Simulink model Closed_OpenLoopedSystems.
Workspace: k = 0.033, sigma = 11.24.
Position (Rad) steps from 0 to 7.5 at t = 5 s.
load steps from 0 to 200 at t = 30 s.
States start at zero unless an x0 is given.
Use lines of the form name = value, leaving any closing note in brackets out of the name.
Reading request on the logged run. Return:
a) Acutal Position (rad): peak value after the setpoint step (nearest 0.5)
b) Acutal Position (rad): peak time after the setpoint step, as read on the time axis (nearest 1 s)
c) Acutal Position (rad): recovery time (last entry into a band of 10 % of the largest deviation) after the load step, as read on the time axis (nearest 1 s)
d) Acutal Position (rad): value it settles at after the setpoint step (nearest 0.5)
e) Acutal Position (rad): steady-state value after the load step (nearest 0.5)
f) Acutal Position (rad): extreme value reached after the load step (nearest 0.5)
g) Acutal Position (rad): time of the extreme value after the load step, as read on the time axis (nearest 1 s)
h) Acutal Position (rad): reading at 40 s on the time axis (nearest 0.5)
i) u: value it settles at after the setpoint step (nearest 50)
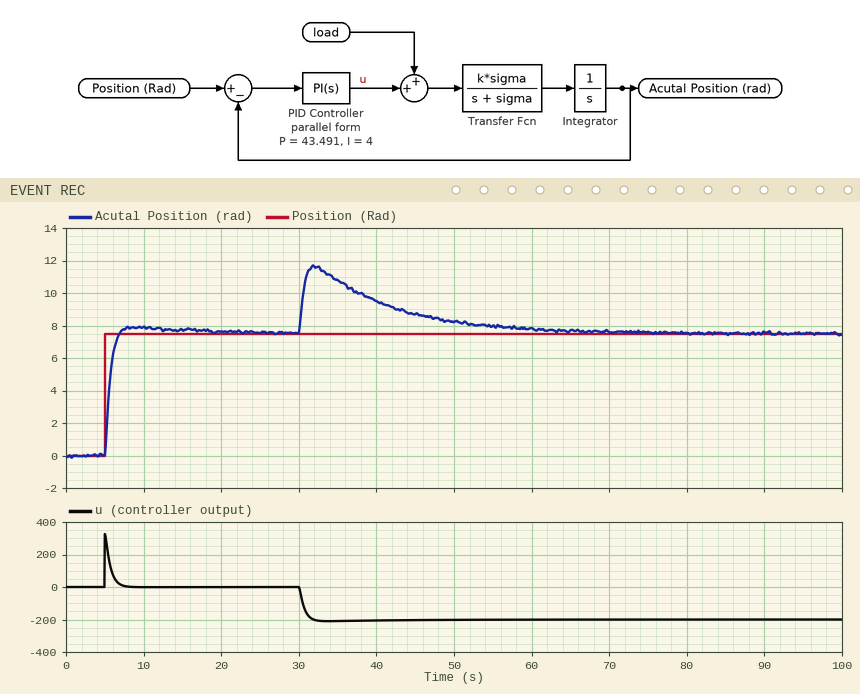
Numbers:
Acutal Position (rad): peak value after the setpoint step = 8.0
Acutal Position (rad): peak time after the setpoint step, as read on the time axis = 9 s
Acutal Position (rad): recovery time (last entry into a band of 10 % of the largest deviation) after the load step, as read on the time axis = 56 s
Acutal Position (rad): value it settles at after the setpoint step = 7.5
Acutal Position (rad): steady-state value after the load step = 7.5
Acutal Position (rad): extreme value reached after the load step = 11.5
Acutal Position (rad): time of the extreme value after the load step, as read on the time axis = 32 s
Acutal Position (rad): reading at 40 s on the time axis = 9.5
u: value it settles at after the setpoint step = 0
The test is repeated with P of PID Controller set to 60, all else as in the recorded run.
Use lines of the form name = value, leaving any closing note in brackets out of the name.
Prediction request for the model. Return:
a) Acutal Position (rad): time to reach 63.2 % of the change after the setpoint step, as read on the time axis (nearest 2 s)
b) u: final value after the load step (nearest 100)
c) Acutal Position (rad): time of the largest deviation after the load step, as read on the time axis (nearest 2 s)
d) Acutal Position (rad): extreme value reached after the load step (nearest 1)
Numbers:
Acutal Position (rad): time to reach 63.2 % of the change after the setpoint step, as read on the time axis = 6 s
u: final value after the load step = -200
Acutal Position (rad): time of the largest deviation after the load step, as read on the time axis = 32 s
Acutal Position (rad): extreme value reached after the load step = 11
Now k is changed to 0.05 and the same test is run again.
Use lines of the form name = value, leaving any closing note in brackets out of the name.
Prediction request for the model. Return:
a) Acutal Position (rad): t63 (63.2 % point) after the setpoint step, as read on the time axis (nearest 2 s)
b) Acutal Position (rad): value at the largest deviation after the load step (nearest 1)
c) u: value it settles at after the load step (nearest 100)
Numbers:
Acutal Position (rad): t63 (63.2 % point) after the setpoint step, as read on the time axis = 6 s
Acutal Position (rad): value at the largest deviation after the load step = 12
u: value it settles at after the load step = -200
